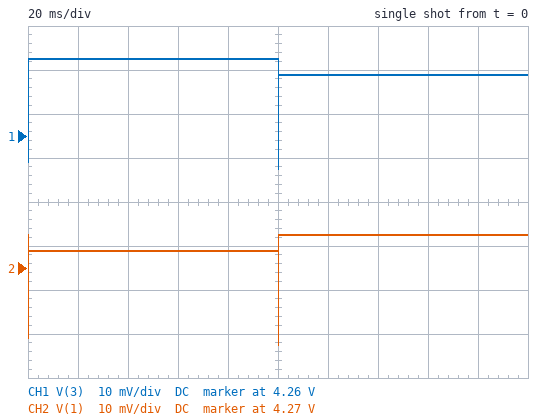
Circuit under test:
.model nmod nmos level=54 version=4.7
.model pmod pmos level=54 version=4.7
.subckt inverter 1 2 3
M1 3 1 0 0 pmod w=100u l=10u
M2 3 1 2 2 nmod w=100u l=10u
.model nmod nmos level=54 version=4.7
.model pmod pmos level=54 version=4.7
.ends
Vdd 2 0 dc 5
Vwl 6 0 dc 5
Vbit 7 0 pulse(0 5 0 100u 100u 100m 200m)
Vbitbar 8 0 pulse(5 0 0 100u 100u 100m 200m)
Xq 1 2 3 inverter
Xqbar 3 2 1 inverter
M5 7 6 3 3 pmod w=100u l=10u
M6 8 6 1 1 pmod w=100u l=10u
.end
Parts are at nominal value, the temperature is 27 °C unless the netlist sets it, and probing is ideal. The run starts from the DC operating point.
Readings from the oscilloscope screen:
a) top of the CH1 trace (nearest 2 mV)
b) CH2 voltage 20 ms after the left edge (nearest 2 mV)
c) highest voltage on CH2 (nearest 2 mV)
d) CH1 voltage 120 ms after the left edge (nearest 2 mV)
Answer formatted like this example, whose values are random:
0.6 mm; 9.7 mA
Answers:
4.278 V; 4.274 V; 4.278 V; 4.274 V
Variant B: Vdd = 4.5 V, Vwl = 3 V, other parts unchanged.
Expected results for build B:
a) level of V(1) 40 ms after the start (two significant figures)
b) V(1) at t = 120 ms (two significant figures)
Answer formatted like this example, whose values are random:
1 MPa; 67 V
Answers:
4.1 V; 4.8 V
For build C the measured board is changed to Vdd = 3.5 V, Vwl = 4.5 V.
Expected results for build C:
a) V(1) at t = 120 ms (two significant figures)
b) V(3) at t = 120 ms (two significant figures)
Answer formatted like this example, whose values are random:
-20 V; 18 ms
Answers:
4.0 V; 3.5 V
